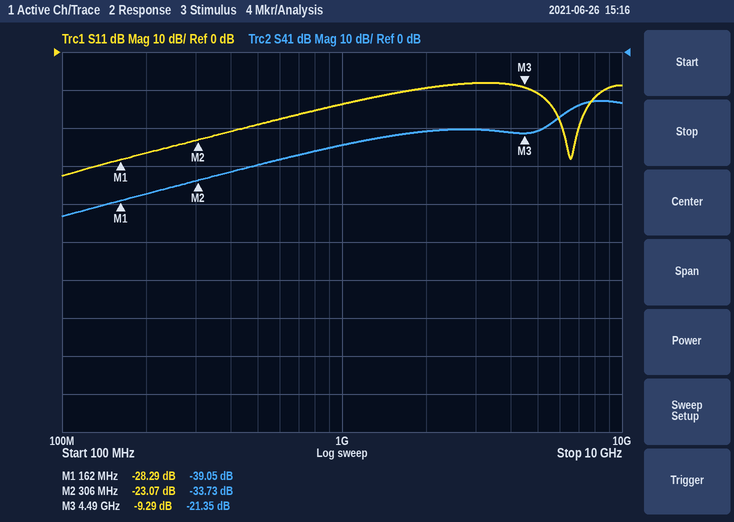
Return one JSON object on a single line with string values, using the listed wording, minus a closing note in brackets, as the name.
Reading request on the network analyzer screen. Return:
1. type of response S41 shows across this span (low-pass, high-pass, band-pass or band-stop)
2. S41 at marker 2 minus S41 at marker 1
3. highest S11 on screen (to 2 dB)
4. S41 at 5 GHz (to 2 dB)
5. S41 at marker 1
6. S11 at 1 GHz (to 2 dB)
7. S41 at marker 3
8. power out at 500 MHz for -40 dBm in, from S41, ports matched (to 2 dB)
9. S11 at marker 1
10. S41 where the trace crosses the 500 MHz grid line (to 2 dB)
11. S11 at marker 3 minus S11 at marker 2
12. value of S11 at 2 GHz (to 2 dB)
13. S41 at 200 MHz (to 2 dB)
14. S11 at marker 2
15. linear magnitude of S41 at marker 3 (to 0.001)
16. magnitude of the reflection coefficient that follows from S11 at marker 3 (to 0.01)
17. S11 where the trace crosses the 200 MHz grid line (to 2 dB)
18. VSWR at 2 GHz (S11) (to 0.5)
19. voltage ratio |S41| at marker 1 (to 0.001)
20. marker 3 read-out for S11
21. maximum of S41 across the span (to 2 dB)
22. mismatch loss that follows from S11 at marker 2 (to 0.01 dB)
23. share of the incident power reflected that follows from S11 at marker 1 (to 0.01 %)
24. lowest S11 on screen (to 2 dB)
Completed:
{"type of response S41 shows across this span": "high-pass", "S41 at marker 2 minus S41 at marker 1": "5.32 dB", "highest S11 on screen": "-8 dB", "S41 at 5 GHz": "-20 dB", "S41 at marker 1": "-39.05 dB", "S11 at 1 GHz": "-14 dB", "S41 at marker 3": "-21.35 dB", "power out at 500 MHz for -40 dBm in, from S41, ports matched": "-70 dBm", "S11 at marker 1": "-28.29 dB", "S41 where the trace crosses the 500 MHz grid line": "-30 dB", "S11 at marker 3 minus S11 at marker 2": "13.78 dB", "value of S11 at 2 GHz": "-10 dB", "S41 at 200 MHz": "-38 dB", "S11 at marker 2": "-23.07 dB", "linear magnitude of S41 at marker 3": "0.086", "magnitude of the reflection coefficient that follows from S11 at marker 3": "0.34", "S11 where the trace crosses the 200 MHz grid line": "-26 dB", "VSWR at 2 GHz (S11)": "2.0", "voltage ratio |S41| at marker 1": "0.011", "marker 3 read-out for S11": "-9.29 dB", "maximum of S41 across the span": "-12 dB", "mismatch loss that follows from S11 at marker 2": "0.02 dB", "share of the incident power reflected that follows from S11 at marker 1": "0.15 %", "lowest S11 on screen": "-32 dB"}
